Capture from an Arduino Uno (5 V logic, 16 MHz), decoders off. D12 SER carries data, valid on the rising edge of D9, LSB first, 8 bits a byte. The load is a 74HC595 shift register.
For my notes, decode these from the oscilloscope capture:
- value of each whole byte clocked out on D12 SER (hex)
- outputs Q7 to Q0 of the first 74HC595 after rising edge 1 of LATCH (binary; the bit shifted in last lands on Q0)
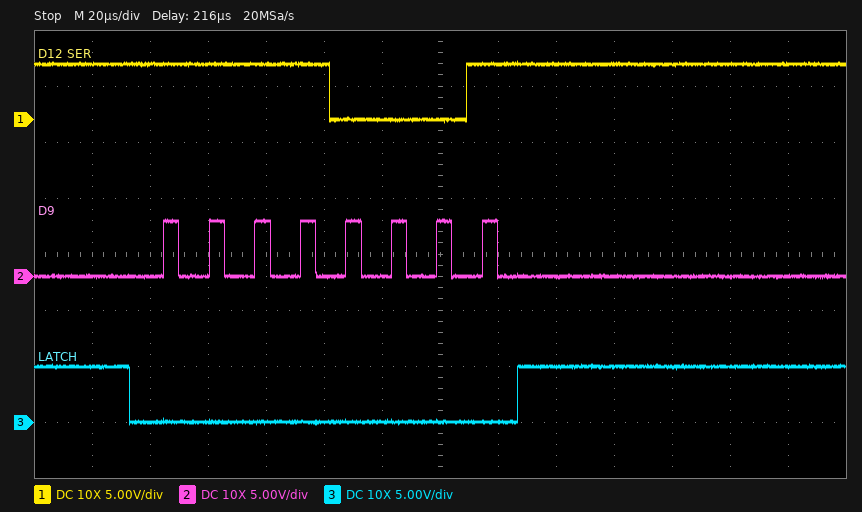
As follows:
8F
11110001
